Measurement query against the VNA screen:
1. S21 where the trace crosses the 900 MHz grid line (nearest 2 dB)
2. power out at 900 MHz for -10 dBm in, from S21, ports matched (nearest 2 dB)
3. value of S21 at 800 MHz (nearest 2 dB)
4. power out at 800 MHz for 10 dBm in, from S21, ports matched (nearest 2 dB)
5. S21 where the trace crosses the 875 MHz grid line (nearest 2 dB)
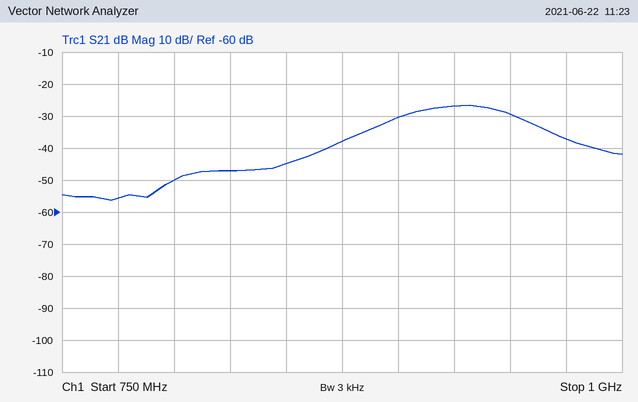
-30 dB
-40 dBm
-50 dB
-40 dBm
-38 dB
